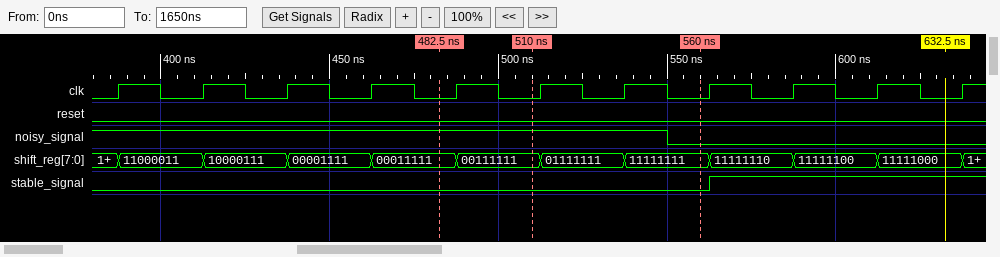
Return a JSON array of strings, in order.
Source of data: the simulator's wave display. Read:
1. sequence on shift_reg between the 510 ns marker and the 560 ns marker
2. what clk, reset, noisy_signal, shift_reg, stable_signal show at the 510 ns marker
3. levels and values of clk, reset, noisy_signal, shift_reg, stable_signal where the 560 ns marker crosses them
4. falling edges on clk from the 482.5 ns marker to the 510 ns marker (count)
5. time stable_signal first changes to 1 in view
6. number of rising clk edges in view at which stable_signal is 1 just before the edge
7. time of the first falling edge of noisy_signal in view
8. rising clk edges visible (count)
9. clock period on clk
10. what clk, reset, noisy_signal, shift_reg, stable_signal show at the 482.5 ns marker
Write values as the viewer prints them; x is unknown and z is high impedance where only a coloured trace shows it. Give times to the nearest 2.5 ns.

["00111111, 01111111, 11111111", "clk=0, reset=0, noisy_signal=1, shift_reg=00111111, stable_signal=0", "clk=0, reset=0, noisy_signal=0, shift_reg=11111111, stable_signal=0", "1", "562.5 ns", "3", "550 ns", "11", "25 ns", "clk=0, reset=0, noisy_signal=1, shift_reg=00011111, stable_signal=0"]
